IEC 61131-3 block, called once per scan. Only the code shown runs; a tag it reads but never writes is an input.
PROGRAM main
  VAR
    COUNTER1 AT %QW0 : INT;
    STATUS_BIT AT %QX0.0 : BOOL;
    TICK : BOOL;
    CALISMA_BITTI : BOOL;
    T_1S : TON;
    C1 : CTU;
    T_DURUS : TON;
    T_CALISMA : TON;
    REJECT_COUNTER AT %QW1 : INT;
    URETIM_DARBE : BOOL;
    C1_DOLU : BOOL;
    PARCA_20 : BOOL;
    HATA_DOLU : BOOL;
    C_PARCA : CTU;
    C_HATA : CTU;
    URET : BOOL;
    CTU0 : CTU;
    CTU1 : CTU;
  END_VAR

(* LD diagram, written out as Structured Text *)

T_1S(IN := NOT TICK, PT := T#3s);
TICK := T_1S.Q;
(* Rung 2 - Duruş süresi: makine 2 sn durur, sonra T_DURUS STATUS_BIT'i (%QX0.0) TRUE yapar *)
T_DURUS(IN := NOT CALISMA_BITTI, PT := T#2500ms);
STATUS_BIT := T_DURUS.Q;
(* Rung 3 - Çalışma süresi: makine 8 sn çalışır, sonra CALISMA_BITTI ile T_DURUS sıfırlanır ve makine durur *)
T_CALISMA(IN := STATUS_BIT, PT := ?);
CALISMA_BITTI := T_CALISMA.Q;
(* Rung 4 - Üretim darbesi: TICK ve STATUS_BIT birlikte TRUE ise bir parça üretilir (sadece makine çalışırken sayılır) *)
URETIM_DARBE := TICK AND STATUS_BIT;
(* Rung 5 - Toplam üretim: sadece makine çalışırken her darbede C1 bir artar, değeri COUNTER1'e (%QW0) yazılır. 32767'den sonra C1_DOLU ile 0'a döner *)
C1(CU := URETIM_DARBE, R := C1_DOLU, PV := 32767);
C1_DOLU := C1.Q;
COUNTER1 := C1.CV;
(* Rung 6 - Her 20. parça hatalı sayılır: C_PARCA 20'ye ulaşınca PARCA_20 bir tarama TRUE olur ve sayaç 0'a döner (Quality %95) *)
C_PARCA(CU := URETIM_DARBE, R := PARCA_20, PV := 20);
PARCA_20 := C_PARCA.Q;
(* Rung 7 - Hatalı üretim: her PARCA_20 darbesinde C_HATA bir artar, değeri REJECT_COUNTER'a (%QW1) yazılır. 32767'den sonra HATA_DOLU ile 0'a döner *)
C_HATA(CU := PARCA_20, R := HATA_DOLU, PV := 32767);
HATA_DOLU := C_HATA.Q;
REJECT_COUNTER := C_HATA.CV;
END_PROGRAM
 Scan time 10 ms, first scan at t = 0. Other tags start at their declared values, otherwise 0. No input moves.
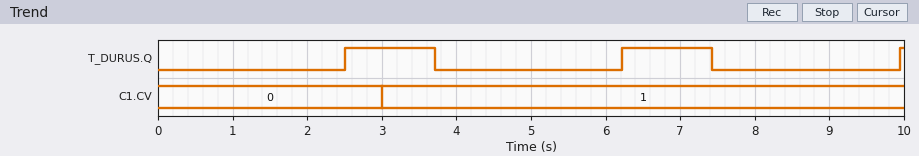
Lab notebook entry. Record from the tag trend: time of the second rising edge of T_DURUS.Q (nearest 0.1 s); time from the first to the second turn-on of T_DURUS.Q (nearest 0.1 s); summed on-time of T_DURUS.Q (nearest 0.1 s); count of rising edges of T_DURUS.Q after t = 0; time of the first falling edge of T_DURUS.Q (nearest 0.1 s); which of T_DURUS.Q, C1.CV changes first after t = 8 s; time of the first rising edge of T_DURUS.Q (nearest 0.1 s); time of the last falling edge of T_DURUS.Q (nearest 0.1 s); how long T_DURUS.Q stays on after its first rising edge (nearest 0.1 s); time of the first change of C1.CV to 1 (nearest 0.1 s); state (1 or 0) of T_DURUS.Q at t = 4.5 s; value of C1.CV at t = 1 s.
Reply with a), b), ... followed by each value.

a) 6.2 s
b) 3.7 s
c) 2.5 s
d) 3
e) 3.7 s
f) T_DURUS.Q
g) 2.5 s
h) 7.4 s
i) 1.2 s
j) 3.0 s
k) 0
l) 0
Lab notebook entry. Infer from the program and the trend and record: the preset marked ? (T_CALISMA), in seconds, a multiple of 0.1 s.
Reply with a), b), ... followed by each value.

a) 1.2 s
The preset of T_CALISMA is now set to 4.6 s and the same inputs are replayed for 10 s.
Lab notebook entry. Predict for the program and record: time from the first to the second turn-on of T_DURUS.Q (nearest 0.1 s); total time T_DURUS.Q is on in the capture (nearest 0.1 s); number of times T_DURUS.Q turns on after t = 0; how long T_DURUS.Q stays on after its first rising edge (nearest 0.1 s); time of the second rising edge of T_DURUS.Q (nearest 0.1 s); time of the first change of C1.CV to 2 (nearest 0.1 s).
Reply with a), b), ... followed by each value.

a) 7.1 s
b) 5.0 s
c) 2
d) 4.6 s
e) 9.6 s
f) 6.0 s
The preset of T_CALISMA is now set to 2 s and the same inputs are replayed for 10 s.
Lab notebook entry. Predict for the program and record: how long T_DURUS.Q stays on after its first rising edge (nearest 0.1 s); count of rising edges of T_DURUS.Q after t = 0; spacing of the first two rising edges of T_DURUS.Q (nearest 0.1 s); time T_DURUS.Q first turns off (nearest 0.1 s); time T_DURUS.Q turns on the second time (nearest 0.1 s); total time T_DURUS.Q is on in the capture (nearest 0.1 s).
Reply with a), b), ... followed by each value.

a) 2.0 s
b) 2
c) 4.5 s
d) 4.5 s
e) 7.0 s
f) 4.0 s
